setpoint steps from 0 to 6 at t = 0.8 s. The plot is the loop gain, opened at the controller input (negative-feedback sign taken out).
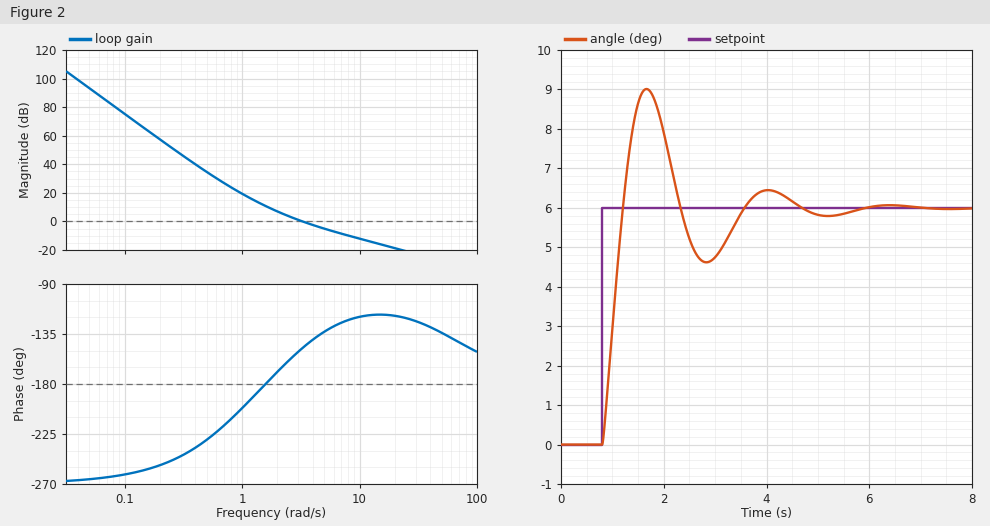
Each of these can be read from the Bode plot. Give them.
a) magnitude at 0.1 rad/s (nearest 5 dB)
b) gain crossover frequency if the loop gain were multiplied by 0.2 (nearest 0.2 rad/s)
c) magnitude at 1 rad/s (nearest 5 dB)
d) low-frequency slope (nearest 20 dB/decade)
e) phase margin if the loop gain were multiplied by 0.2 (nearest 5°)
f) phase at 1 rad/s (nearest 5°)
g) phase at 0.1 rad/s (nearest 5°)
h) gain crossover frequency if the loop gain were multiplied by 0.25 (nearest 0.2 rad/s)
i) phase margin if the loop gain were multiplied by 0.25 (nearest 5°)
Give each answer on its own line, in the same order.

75 dB
1.4 rad/s
20 dB
-60 dB/decade
-10°
-200°
-260°
1.4 rad/s
-5°
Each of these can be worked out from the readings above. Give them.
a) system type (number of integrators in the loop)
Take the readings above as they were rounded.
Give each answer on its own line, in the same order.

3
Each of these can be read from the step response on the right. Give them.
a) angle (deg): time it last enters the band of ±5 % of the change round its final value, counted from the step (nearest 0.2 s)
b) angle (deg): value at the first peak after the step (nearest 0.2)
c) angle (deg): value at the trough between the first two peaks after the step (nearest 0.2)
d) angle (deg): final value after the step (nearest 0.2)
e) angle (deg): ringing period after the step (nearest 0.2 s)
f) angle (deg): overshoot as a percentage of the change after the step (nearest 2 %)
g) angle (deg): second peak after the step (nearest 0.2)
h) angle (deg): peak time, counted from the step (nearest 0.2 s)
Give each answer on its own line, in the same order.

3.6 s
9.0
4.6
6.0
2.4 s
50 %
6.4
0.8 s
